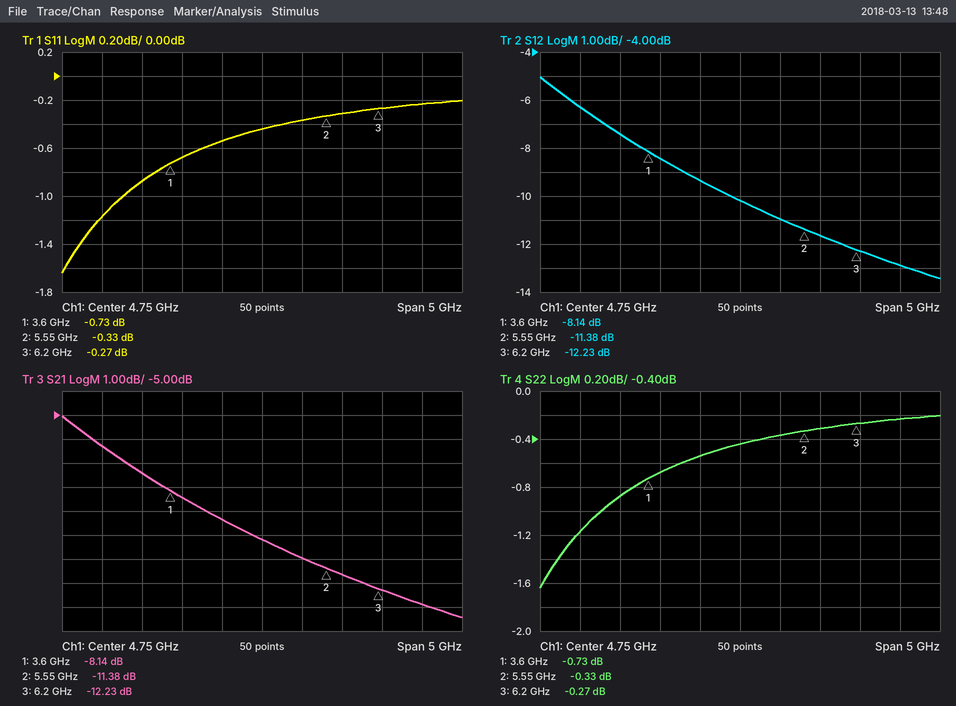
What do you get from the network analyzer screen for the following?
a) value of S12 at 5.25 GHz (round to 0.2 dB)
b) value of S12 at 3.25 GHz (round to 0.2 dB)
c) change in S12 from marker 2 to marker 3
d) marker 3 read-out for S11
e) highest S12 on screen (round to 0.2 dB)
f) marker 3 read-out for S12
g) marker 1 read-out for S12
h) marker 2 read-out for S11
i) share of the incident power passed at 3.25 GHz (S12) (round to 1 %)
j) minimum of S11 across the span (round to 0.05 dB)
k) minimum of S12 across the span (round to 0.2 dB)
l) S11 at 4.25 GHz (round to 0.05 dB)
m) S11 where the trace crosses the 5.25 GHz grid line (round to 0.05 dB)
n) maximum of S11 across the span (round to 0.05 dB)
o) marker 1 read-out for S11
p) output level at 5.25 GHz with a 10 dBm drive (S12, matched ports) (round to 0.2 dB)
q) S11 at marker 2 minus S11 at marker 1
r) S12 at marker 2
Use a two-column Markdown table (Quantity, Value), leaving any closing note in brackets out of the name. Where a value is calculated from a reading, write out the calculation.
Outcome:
| Quantity | Value |
|---|---|
| value of S12 at 5.25 GHz | -11.0 dB |
| value of S12 at 3.25 GHz | -7.4 dB |
| change in S12 from marker 2 to marker 3 | -12.23 − (-11.38) = -0.85 dB |
| marker 3 read-out for S11 | -0.27 dB |
| highest S12 on screen | -5.0 dB |
| marker 3 read-out for S12 | -12.23 dB |
| marker 1 read-out for S12 | -8.14 dB |
| marker 2 read-out for S11 | -0.33 dB |
| share of the incident power passed at 3.25 GHz (S12) | 10^(-7.4/10) ≈ 18 % |
| minimum of S11 across the span | -1.65 dB |
| minimum of S12 across the span | -13.4 dB |
| S11 at 4.25 GHz | -0.55 dB |
| S11 where the trace crosses the 5.25 GHz grid line | -0.35 dB |
| maximum of S11 across the span | -0.20 dB |
| marker 1 read-out for S11 | -0.73 dB |
| output level at 5.25 GHz with a 10 dBm drive (S12, matched ports) | 10 dBm + (-11.0 dB) = -1.0 dBm |
| S11 at marker 2 minus S11 at marker 1 | -0.33 − (-0.73) = 0.40 dB |
| S12 at marker 2 | -11.38 dB |
